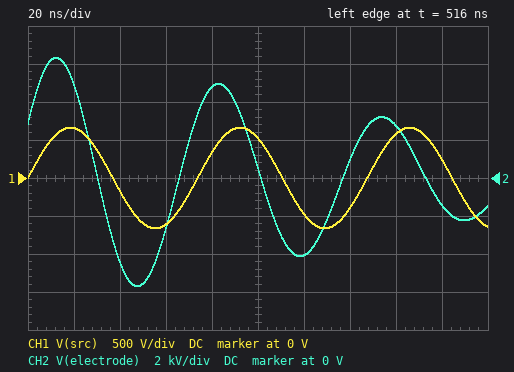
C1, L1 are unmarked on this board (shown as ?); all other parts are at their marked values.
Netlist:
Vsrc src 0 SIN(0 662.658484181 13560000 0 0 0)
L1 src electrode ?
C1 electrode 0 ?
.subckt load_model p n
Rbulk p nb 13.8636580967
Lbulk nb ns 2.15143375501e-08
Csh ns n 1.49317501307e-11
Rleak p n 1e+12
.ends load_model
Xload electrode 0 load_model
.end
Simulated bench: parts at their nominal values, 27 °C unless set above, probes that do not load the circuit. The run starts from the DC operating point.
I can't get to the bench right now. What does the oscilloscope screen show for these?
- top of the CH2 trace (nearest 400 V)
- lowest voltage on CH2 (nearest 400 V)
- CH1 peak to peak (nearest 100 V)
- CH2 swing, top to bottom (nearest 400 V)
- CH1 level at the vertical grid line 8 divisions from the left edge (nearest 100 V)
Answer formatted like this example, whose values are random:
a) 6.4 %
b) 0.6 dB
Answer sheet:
a) 6.4 kV
b) -5.6 kV
c) 1.3 kV
d) 12.0 kV
e) 600 V
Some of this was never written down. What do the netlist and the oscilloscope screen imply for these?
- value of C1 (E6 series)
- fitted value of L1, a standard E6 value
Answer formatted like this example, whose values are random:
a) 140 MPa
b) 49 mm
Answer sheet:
a) 100 pF
b) 1 µH
